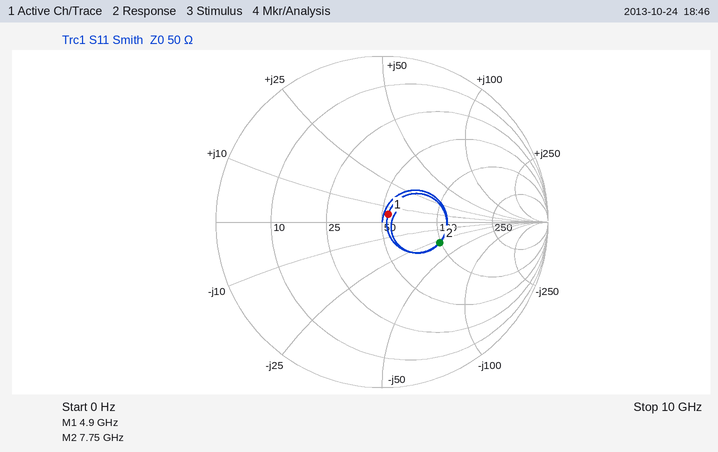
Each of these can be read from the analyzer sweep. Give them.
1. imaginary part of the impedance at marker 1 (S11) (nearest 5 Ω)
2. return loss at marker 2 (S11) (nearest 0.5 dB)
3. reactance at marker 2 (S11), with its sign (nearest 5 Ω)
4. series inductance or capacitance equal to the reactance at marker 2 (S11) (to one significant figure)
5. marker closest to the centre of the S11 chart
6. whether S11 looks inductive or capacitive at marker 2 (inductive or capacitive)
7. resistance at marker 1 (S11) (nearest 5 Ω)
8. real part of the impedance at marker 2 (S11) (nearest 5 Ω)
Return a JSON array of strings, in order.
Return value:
["+5 Ω", "8.5 dB", "-30 Ω", "700 fF", "marker 1", "capacitive", "55 Ω", "100 Ω"]
